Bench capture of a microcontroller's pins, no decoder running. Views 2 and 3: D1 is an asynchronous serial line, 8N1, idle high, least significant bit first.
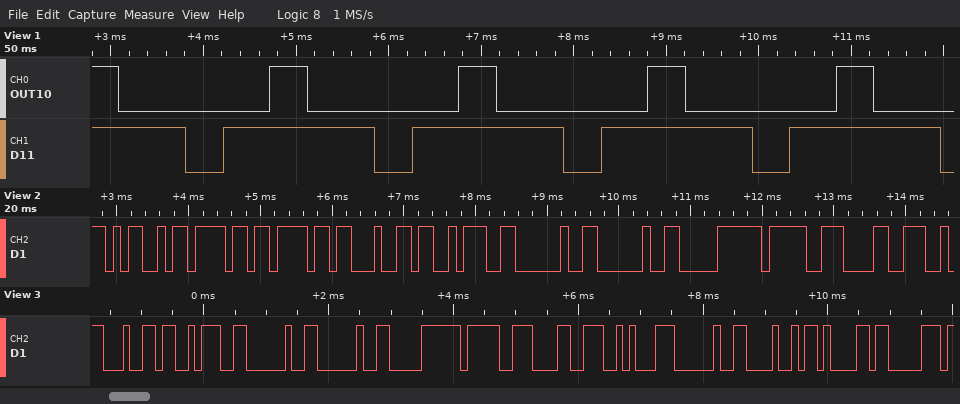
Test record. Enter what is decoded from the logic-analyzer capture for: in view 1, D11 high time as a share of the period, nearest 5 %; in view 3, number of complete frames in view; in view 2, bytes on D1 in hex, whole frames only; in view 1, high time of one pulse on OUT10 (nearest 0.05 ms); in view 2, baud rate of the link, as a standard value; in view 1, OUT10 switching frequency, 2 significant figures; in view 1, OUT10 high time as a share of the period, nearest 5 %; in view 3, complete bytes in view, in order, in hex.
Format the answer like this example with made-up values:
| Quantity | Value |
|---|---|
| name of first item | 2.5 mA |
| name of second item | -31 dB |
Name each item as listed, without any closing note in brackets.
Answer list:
| Quantity | Value |
|---|---|
| in view 1, D11 high time as a share of the period, nearest 5 % | 80 % |
| in view 3, number of complete frames in view | 12 |
| in view 2, bytes on D1 in hex, whole frames only | 0x4D 0x6F 0x6F 0x64 0x3A 0x20 0x20 0xF0 0x9F 0x98 |
| in view 1, high time of one pulse on OUT10 | 0.40 ms |
| in view 2, baud rate of the link, as a standard value | 9600 baud |
| in view 1, OUT10 switching frequency, 2 significant figures | 490 Hz |
| in view 1, OUT10 high time as a share of the period, nearest 5 % | 20 % |
| in view 3, complete bytes in view, in order, in hex | 0x64 0x3A 0x20 0x20 0xF0 0x9F 0x98 0x8A 0x20 0x48 0x61 0x70 |
